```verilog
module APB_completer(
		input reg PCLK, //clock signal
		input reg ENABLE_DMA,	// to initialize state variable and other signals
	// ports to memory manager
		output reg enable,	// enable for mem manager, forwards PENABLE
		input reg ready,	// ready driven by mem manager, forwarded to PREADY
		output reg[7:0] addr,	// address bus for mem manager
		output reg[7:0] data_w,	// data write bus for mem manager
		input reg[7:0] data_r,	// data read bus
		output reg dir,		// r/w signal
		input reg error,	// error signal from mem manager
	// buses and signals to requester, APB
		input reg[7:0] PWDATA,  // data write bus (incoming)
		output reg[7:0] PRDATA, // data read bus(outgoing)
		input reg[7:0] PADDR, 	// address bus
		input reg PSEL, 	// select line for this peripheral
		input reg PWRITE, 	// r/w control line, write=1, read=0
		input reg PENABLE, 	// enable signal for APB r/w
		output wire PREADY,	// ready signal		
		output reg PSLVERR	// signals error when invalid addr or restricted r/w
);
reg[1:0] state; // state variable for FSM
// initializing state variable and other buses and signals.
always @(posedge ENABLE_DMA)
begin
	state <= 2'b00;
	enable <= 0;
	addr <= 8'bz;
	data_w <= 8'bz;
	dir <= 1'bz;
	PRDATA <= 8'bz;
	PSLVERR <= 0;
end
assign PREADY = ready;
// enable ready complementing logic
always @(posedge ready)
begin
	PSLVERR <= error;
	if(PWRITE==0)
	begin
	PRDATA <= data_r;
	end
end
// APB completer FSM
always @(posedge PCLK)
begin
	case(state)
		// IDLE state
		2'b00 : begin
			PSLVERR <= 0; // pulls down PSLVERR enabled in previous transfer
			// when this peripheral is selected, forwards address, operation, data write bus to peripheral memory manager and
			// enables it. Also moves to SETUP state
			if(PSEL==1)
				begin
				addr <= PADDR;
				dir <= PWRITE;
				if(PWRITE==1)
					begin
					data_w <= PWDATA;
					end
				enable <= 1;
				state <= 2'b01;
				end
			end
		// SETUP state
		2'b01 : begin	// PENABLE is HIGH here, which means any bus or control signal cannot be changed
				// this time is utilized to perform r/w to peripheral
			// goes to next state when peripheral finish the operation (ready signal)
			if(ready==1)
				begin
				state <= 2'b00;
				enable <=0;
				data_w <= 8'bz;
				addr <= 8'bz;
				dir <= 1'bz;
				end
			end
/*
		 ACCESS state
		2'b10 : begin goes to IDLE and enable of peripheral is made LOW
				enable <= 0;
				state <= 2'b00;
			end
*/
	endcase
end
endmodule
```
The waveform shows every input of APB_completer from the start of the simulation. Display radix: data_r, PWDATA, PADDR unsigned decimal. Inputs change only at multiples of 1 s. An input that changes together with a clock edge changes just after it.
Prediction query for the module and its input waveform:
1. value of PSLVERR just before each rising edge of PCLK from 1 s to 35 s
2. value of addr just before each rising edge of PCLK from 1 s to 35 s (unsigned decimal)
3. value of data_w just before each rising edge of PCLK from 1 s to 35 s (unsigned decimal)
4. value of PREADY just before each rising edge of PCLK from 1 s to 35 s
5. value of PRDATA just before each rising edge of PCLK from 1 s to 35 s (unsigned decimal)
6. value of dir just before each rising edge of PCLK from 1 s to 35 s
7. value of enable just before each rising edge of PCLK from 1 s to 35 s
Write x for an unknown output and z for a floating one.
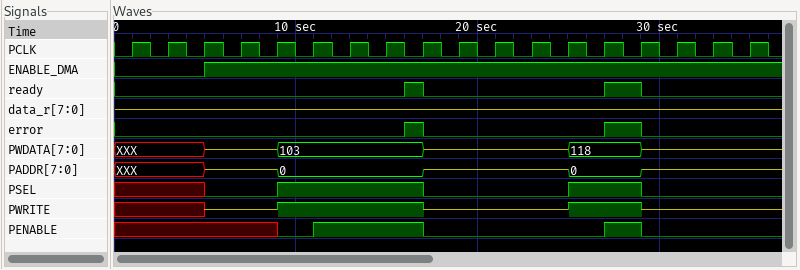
x x x 0 0 0 0 0 1 1 0 0 0 0 1 1 0 0
x, x, x, z, z, z, 0, 0, 0, z, z, z, z, z, 0, z, z, z
x, x, x, z, z, z, 103, 103, 103, z, z, z, z, z, 118, z, z, z
0 0 0 0 0 0 0 0 1 0 0 0 0 0 1 0 0 0
x, x, x, z, z, z, z, z, z, z, z, z, z, z, z, z, z, z
x x x z z z 1 1 1 z z z z z 1 z z z
x x x 0 0 0 1 1 1 0 0 0 0 0 1 0 0 0
